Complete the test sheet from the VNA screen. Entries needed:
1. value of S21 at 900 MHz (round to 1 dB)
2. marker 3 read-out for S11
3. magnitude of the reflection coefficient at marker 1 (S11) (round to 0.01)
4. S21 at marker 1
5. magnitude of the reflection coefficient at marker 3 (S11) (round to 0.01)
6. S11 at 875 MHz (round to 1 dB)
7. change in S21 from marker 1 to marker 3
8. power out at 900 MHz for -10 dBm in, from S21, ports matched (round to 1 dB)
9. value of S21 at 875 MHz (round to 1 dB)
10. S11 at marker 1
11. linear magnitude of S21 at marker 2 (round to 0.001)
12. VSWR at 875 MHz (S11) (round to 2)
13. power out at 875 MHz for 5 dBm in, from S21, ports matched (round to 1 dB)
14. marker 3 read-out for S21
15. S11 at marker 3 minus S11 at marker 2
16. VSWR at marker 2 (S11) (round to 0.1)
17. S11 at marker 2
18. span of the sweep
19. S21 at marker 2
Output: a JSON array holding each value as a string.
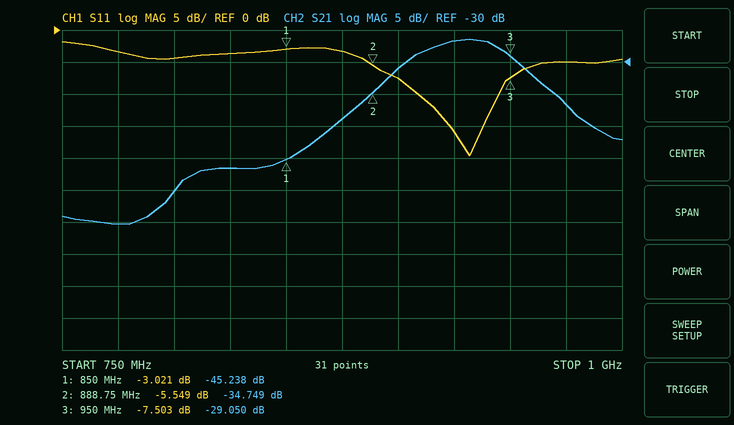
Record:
["-31 dB", "-7.503 dB", "0.71", "-45.238 dB", "0.42", "-3 dB", "16.188 dB", "-41 dBm", "-39 dB", "-3.021 dB", "0.018", "6", "-34 dBm", "-29.050 dB", "-1.954 dB", "3.2", "-5.549 dB", "250 MHz", "-34.749 dB"]
